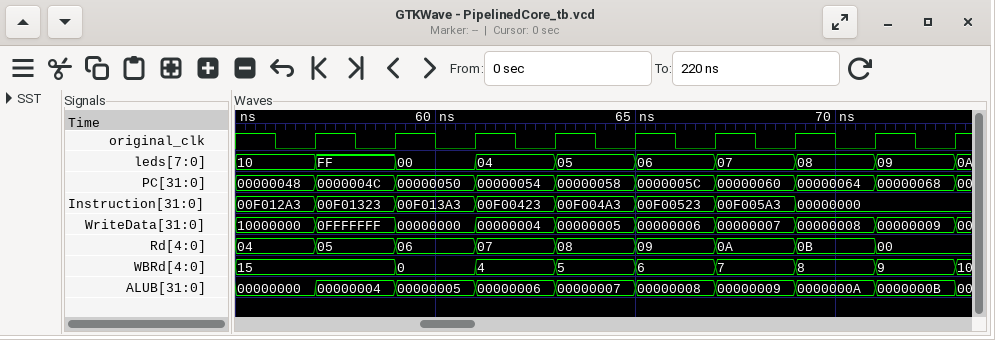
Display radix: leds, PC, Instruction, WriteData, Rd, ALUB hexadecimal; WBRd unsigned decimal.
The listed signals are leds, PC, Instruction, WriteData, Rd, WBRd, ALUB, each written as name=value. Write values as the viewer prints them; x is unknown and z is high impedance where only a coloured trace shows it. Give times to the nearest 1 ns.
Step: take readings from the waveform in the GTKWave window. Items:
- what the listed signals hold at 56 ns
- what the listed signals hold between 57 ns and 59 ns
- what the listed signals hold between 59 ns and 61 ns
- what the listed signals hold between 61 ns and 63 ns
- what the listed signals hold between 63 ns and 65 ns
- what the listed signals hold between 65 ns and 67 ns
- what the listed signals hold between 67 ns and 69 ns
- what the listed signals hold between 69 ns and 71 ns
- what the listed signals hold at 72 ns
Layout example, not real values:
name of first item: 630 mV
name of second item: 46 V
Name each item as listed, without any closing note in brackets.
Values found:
what the listed signals hold at 56 ns: leds=10, PC=00000048, Instruction=00F012A3, WriteData=10000000, Rd=04, WBRd=15, ALUB=00000000
what the listed signals hold between 57 ns and 59 ns: leds=FF, PC=0000004C, Instruction=00F01323, WriteData=0FFFFFFF, Rd=05, WBRd=15, ALUB=00000004
what the listed signals hold between 59 ns and 61 ns: leds=00, PC=00000050, Instruction=00F013A3, WriteData=00000000, Rd=06, WBRd=0, ALUB=00000005
what the listed signals hold between 61 ns and 63 ns: leds=04, PC=00000054, Instruction=00F00423, WriteData=00000004, Rd=07, WBRd=4, ALUB=00000006
what the listed signals hold between 63 ns and 65 ns: leds=05, PC=00000058, Instruction=00F004A3, WriteData=00000005, Rd=08, WBRd=5, ALUB=00000007
what the listed signals hold between 65 ns and 67 ns: leds=06, PC=0000005C, Instruction=00F00523, WriteData=00000006, Rd=09, WBRd=6, ALUB=00000008
what the listed signals hold between 67 ns and 69 ns: leds=07, PC=00000060, Instruction=00F005A3, WriteData=00000007, Rd=0A, WBRd=7, ALUB=00000009
what the listed signals hold between 69 ns and 71 ns: leds=08, PC=00000064, Instruction=00000000, WriteData=00000008, Rd=0B, WBRd=8, ALUB=0000000A
what the listed signals hold at 72 ns: leds=09, PC=00000068, Instruction=00000000, WriteData=00000009, Rd=00, WBRd=9, ALUB=0000000B
